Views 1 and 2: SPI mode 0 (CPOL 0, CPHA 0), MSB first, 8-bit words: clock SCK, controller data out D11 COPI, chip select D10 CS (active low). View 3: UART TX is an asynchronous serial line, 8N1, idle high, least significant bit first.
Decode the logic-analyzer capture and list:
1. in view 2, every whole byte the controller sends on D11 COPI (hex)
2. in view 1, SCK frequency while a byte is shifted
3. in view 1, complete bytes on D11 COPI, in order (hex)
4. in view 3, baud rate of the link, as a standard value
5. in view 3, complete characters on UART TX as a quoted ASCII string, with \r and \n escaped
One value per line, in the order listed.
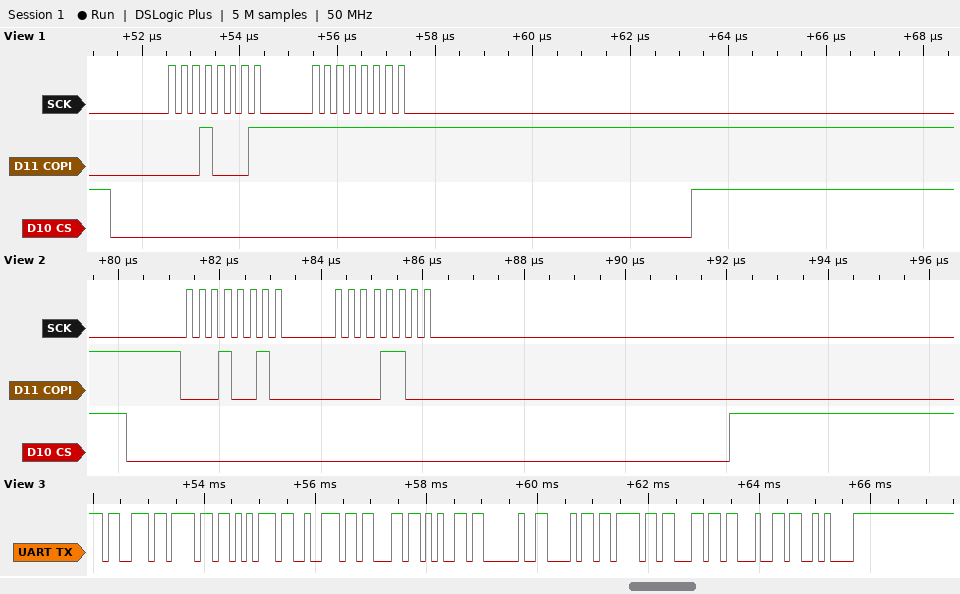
0x12 0x0C
4 MHz
0x11 0xFF
9600 baud
"source hold\n"
